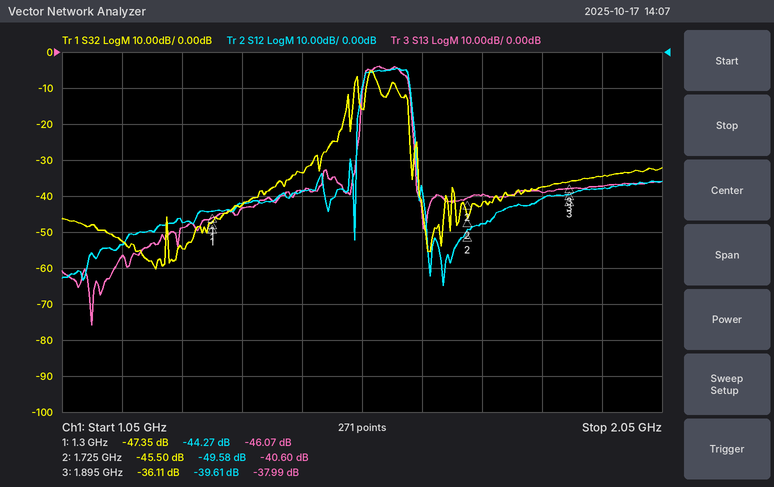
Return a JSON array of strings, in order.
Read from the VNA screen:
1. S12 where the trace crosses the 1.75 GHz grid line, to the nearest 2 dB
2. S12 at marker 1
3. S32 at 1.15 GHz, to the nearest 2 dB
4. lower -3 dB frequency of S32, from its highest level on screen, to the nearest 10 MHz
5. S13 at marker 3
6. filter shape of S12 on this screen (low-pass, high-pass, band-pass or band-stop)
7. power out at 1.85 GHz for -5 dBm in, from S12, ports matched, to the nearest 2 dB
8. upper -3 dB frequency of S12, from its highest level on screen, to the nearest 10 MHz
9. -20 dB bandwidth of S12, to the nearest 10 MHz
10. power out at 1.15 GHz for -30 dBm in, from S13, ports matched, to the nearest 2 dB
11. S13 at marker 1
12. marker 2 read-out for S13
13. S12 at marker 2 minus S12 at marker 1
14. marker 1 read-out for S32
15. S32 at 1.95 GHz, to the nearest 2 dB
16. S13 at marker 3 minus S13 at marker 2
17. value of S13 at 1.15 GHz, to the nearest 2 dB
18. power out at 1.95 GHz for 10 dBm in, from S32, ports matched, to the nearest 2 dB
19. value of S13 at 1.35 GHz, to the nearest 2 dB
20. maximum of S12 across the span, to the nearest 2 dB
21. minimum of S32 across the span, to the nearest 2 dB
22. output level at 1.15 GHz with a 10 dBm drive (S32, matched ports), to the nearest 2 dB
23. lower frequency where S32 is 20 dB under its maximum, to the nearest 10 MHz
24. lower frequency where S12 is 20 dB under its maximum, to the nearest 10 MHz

["-48 dB", "-44.27 dB", "-52 dB", "1.56 GHz", "-37.99 dB", "band-pass", "-46 dBm", "1.63 GHz", "100 MHz", "-86 dBm", "-46.07 dB", "-40.60 dB", "-5.31 dB", "-47.35 dB", "-34 dB", "2.61 dB", "-56 dB", "-24 dBm", "-44 dB", "-4 dB", "-60 dB", "-42 dBm", "1.50 GHz", "1.54 GHz"]
